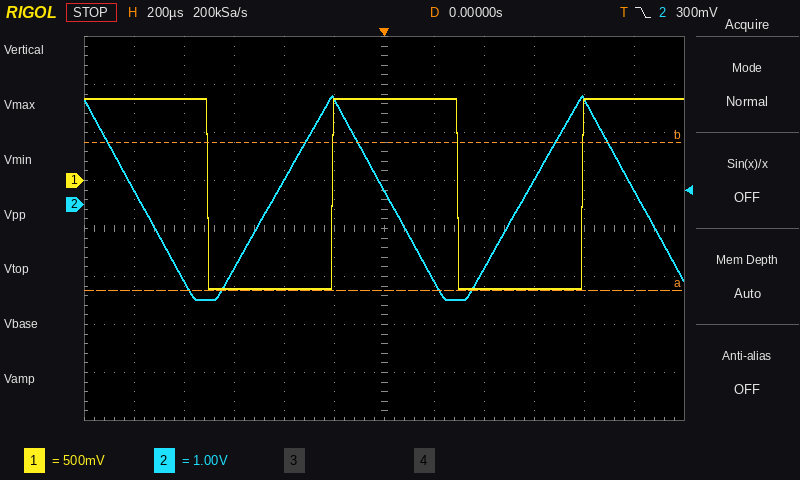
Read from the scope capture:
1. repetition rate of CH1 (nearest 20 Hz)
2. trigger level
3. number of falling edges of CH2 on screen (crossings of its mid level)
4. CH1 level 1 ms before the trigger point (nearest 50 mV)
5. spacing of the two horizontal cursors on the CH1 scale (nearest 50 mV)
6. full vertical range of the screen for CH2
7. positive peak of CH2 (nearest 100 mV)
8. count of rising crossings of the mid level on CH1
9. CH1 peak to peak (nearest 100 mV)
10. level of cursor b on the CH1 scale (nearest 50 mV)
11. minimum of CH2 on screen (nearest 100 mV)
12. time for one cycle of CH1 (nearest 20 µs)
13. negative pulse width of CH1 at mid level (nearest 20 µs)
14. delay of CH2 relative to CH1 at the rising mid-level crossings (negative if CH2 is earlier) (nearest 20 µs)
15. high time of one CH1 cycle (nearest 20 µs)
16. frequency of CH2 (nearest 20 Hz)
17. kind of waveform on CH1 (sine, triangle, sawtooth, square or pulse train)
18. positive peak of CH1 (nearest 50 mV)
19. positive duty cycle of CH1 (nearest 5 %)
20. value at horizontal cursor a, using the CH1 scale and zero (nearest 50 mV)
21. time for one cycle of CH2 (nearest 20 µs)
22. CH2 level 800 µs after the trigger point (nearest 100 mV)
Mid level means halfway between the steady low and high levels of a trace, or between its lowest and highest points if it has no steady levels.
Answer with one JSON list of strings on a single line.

["1.00 kHz", "300 mV", "3", "850 mV", "1.55 V", "8 V", "2.3 V", "2", "2.00 V", "400 mV", "-2.0 V", "1.00 ms", "500 µs", "-240 µs", "500 µs", "1.00 kHz", "square", "850 mV", "50 %", "-1.15 V", "1.00 ms", "2.2 V"]
